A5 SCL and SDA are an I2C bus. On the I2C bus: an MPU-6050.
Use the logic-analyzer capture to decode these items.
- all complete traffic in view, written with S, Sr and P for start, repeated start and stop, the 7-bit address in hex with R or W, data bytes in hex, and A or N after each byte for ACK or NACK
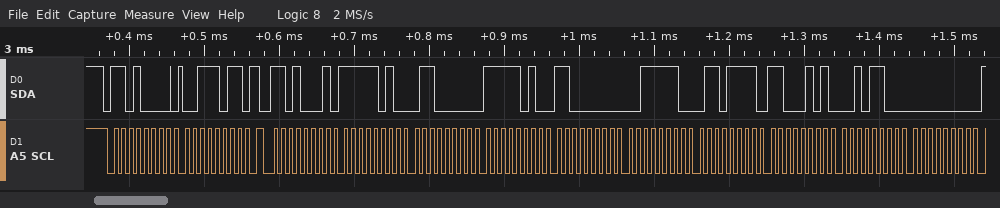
S 68W A 3B A Sr 68R A FA A 60 A FA A C0 A 3E A 6F A C5 A 2C A 00 A
